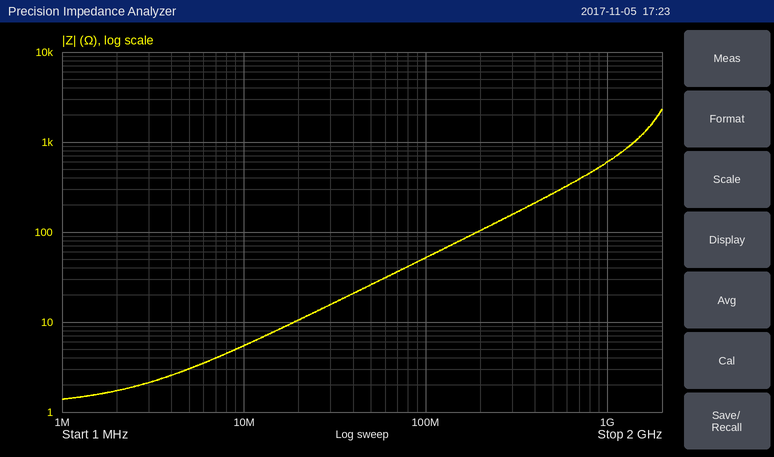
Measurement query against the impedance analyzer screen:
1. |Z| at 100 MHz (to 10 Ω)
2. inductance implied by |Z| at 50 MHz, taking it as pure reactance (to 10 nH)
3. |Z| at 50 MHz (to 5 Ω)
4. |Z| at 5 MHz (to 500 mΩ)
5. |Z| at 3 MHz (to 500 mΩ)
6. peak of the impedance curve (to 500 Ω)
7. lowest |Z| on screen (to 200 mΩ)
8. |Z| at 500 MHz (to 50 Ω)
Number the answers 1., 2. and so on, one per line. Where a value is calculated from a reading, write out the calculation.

1. 50 Ω
2. L = 25 Ω/(2π × 50 MHz) ≈ 80 nH
3. 25 Ω
4. 3.0 Ω
5. 2.0 Ω
6. 2.5 kΩ
7. 1.4 Ω
8. 250 Ω
